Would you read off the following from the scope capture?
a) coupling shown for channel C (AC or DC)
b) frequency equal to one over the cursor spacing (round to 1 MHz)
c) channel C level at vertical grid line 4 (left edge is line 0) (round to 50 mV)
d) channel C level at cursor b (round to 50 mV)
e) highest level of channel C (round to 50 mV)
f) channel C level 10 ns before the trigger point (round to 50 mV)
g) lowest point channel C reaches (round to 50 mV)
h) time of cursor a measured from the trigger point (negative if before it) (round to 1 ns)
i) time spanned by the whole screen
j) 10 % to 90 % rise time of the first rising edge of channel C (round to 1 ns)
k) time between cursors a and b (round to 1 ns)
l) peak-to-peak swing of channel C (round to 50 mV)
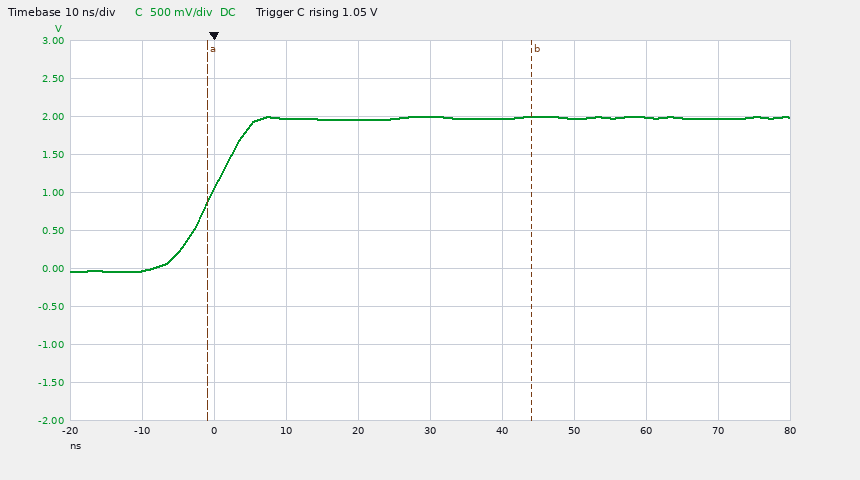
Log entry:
DC
22 MHz
1.95 V
2.00 V
2.00 V
-50 mV
-50 mV
-1 ns
100 ns
10 ns
45 ns
2.05 V
